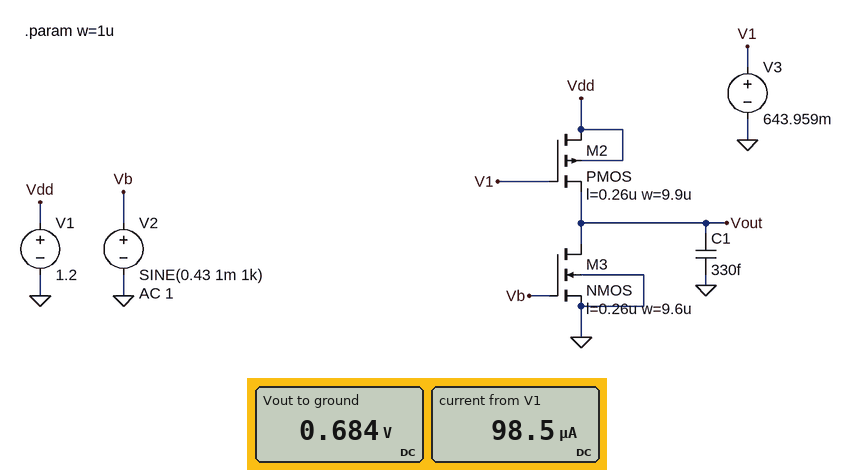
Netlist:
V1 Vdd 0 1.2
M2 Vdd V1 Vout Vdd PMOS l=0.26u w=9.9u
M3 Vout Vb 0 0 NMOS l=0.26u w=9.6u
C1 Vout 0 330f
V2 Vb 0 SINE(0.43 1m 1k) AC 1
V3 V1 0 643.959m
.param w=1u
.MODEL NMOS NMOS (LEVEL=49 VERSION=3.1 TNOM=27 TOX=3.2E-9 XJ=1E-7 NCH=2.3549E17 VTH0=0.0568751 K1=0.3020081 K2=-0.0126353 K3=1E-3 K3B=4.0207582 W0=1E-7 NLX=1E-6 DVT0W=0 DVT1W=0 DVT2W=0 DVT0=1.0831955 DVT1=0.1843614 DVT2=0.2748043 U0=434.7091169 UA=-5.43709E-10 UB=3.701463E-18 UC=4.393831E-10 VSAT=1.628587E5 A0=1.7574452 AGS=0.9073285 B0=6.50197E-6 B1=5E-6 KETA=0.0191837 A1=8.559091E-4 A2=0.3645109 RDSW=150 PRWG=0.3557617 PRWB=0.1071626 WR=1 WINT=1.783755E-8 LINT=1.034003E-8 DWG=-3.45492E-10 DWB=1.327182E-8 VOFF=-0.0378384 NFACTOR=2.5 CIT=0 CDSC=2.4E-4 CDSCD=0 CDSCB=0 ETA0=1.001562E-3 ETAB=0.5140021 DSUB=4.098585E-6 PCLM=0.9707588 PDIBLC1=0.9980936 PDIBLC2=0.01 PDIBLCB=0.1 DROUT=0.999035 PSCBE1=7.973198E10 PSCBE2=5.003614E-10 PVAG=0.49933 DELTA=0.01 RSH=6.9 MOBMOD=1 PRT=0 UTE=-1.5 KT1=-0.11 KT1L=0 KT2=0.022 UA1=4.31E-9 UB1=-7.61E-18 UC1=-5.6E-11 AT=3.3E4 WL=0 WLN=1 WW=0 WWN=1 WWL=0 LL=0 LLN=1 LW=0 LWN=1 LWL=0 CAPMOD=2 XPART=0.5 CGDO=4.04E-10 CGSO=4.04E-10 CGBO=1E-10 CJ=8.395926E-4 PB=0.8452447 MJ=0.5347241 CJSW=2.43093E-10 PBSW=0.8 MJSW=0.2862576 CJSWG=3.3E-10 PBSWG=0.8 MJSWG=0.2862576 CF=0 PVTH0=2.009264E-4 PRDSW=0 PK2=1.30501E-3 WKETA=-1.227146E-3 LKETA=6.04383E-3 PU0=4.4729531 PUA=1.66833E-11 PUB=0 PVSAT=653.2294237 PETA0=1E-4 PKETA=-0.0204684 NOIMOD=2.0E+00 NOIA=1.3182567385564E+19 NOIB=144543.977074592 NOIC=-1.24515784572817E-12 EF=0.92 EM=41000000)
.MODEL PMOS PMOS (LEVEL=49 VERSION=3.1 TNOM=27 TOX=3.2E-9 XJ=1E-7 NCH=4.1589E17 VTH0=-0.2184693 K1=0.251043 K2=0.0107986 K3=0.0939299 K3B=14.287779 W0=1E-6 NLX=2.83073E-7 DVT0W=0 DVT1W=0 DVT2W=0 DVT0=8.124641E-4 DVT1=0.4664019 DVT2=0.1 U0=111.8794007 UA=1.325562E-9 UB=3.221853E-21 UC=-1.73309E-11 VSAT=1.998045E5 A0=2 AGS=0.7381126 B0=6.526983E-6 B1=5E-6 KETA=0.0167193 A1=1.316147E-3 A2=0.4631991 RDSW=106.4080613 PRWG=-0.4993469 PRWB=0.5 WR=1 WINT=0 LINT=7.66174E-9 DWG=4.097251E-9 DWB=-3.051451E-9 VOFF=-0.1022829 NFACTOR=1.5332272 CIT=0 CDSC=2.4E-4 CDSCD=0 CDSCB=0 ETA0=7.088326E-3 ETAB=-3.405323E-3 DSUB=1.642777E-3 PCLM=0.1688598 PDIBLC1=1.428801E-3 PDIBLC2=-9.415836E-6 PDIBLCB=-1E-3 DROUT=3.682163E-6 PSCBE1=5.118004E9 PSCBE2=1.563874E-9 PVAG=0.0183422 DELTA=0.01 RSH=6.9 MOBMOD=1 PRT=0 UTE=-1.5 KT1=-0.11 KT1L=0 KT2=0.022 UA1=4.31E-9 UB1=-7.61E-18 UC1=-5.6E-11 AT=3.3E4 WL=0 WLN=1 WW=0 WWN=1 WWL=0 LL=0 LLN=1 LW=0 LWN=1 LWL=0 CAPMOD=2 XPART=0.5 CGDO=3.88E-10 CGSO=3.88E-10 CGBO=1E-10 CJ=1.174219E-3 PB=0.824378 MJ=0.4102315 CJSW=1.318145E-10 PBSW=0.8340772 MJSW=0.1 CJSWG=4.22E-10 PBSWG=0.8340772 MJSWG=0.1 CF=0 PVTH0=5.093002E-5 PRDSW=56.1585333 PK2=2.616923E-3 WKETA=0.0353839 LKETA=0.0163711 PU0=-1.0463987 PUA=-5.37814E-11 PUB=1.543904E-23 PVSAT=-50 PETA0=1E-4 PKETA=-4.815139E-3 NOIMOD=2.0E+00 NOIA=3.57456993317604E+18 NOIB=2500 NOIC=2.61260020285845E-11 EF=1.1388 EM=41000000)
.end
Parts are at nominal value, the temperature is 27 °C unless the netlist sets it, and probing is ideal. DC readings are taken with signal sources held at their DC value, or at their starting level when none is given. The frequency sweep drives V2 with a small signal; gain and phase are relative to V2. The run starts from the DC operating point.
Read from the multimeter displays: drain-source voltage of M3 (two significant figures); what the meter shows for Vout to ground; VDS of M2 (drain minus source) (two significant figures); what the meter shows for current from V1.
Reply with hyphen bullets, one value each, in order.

- 680 mV
- 0.684 V
- 520 mV
- 98.5 µA
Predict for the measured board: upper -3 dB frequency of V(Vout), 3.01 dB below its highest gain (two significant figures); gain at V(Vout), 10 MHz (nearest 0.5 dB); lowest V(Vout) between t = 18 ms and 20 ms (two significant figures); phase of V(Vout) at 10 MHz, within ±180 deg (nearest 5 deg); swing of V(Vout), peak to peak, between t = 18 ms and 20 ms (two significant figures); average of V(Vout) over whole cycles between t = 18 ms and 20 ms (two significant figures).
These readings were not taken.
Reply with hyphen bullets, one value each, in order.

- 21 MHz
- 30.5 dB
- 650 mV
- 155 deg
- 76 mV
- 680 mV
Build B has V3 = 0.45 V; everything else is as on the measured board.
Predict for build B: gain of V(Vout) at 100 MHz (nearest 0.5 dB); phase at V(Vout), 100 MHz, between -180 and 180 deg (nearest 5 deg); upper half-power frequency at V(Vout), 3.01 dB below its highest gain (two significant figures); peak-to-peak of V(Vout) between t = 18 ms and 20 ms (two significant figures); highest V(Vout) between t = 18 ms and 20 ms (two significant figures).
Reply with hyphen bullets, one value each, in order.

- 4.5 dB
- 170 deg
- 470 MHz
- 3.4 mV
- 1.1 V
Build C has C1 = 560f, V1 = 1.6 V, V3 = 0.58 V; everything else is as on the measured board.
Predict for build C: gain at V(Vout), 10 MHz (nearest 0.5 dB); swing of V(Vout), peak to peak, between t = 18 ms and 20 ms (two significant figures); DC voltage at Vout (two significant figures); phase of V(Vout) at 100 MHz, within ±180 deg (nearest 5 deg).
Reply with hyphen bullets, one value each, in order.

- 0 dB
- 2.0 mV
- 1.5 V
- 170 deg
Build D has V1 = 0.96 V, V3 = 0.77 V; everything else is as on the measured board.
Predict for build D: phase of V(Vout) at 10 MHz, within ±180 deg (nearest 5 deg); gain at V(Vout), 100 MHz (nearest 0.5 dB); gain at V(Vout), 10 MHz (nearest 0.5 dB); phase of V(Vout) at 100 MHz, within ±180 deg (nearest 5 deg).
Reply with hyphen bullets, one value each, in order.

- 155 deg
- -42.5 dB
- -54.5 dB
- 95 deg
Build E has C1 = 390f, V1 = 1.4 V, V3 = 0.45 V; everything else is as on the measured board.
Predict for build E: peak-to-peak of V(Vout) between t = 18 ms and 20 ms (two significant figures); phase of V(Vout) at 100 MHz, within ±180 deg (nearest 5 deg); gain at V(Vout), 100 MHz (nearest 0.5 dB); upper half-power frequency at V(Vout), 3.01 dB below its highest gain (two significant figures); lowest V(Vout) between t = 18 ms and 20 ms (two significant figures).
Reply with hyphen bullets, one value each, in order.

- 2.2 mV
- 170 deg
- 0.5 dB
- 640 MHz
- 1.3 V
